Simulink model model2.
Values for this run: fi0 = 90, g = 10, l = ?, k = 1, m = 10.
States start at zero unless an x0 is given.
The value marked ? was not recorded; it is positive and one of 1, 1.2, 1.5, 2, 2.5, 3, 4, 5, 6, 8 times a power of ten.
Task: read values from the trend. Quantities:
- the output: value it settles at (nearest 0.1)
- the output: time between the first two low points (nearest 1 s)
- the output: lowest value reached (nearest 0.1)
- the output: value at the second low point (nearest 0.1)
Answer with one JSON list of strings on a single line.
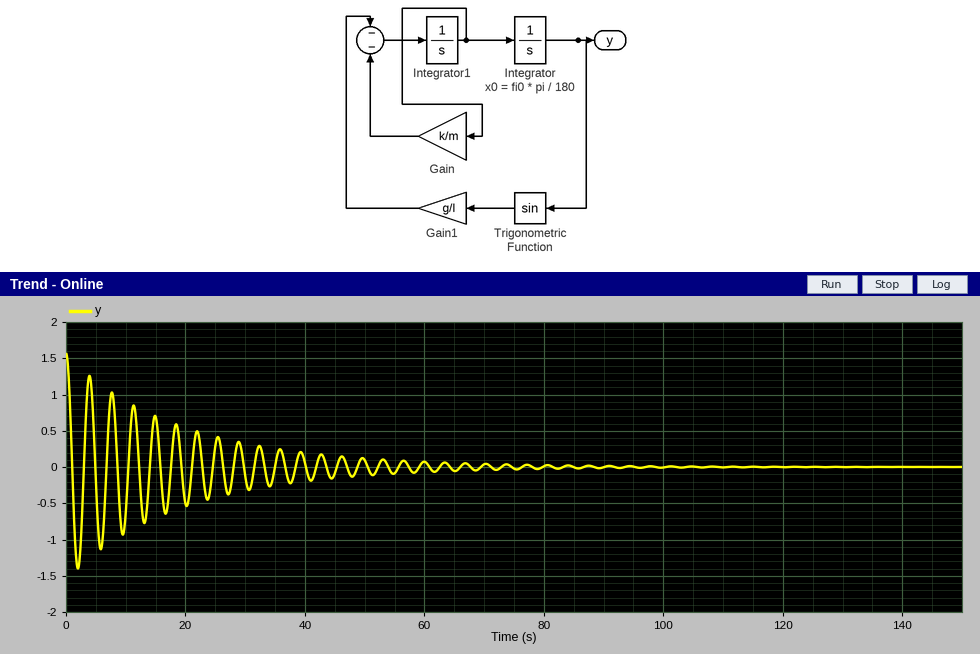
["0.0", "4 s", "-1.4", "-1.1"]
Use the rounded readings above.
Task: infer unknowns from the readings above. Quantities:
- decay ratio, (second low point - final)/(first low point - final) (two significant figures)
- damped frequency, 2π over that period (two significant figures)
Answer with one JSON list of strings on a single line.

["0.79", "1.6 rad/s"]
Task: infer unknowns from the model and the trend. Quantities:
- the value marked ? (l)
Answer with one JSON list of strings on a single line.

["3"]
